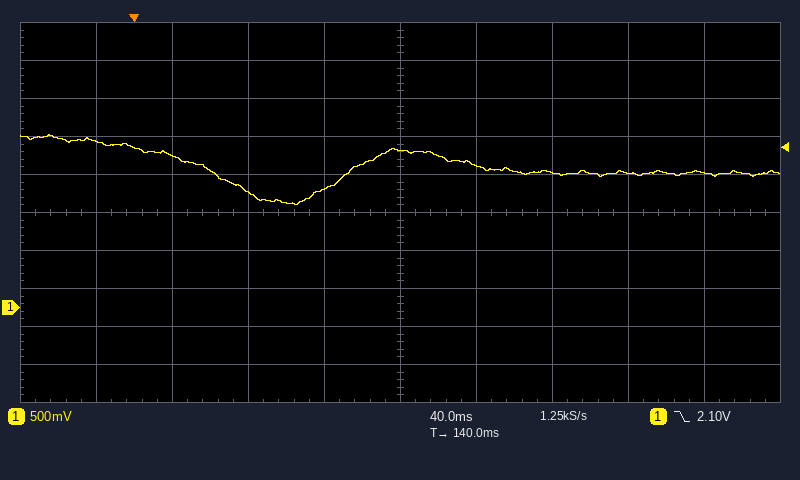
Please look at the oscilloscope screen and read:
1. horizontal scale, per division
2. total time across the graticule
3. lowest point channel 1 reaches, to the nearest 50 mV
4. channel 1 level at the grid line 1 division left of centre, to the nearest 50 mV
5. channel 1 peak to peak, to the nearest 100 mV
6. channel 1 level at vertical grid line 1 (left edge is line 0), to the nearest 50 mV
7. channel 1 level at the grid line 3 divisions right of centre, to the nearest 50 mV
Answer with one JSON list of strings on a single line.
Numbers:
["40 ms", "400 ms", "1.35 V", "1.55 V", "900 mV", "2.20 V", "1.75 V"]
